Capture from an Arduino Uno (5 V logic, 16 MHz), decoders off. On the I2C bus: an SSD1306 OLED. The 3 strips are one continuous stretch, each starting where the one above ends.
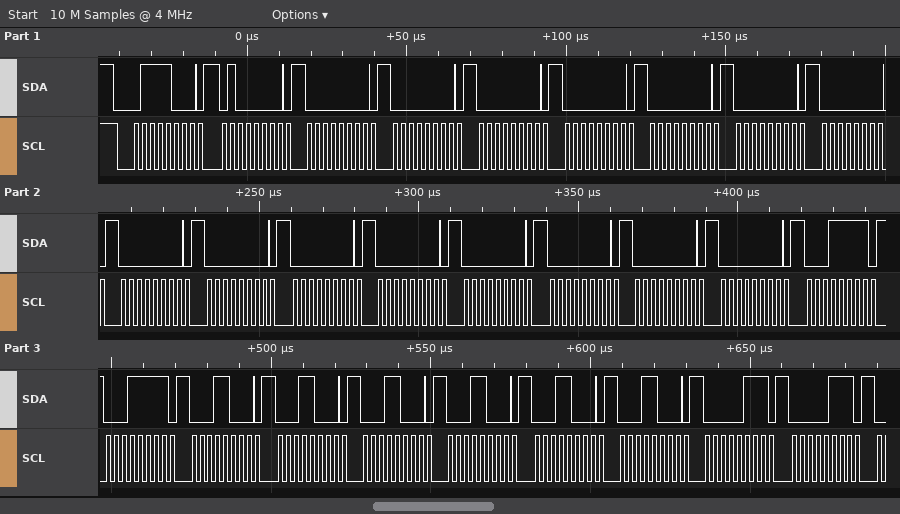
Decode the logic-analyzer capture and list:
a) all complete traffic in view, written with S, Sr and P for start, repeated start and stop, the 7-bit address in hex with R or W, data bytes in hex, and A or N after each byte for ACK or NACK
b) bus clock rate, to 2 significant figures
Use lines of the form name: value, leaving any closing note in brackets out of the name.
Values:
all complete traffic in view, written with S, Sr and P for start, repeated start and stop, the 7-bit address in hex with R or W, data bytes in hex, and A or N after each byte for ACK or NACK: S 3CW A 40 A 00 A 00 A 00 A 00 A 00 A 00 A 00 A 00 A 00 A 00 A 00 A 00 A 00 A 00 A 00 A 1F A 1F A 18 A 18 A 18 A 18 A 18 A 18 A 07 A 07 A
bus clock rate, to 2 significant figures: 400 kHz
